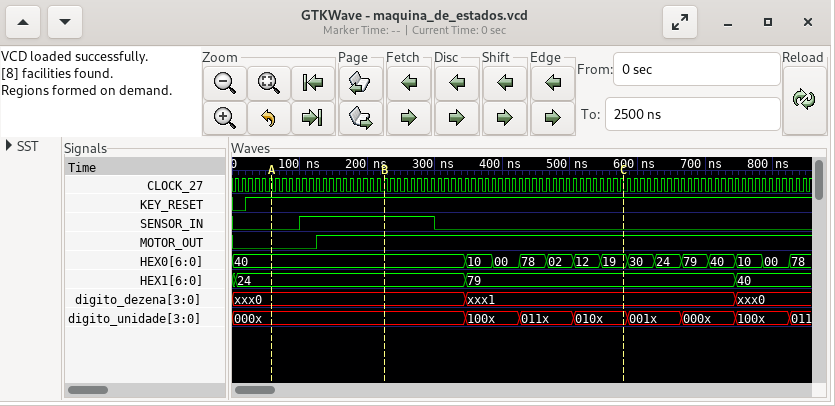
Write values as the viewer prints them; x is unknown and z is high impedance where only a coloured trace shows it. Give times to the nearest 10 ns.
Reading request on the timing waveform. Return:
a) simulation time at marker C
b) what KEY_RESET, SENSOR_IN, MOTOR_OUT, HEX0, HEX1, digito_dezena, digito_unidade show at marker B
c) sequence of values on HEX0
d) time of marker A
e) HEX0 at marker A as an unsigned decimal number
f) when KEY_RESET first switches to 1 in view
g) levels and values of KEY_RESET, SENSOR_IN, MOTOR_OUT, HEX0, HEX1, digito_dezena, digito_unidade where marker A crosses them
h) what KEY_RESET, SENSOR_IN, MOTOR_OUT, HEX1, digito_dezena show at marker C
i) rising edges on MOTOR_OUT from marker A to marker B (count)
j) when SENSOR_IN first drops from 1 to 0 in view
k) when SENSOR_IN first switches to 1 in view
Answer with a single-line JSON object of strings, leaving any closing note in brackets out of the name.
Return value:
{"simulation time at marker C": "580 ns", "what KEY_RESET, SENSOR_IN, MOTOR_OUT, HEX0, HEX1, digito_dezena, digito_unidade show at marker B": "KEY_RESET=1, SENSOR_IN=1, MOTOR_OUT=1, HEX0=40, HEX1=24, digito_dezena=xxx0, digito_unidade=000x", "sequence of values on HEX0": "40, 10, 00, 78, 02, 12, 19, 30, 24, 79, 40, 10, 00, 78", "time of marker A": "60 ns", "HEX0 at marker A as an unsigned decimal number": "64", "when KEY_RESET first switches to 1 in view": "20 ns", "levels and values of KEY_RESET, SENSOR_IN, MOTOR_OUT, HEX0, HEX1, digito_dezena, digito_unidade where marker A crosses them": "KEY_RESET=1, SENSOR_IN=0, MOTOR_OUT=0, HEX0=40, HEX1=24, digito_dezena=xxx0, digito_unidade=000x", "what KEY_RESET, SENSOR_IN, MOTOR_OUT, HEX1, digito_dezena show at marker C": "KEY_RESET=1, SENSOR_IN=0, MOTOR_OUT=1, HEX1=79, digito_dezena=xxx1", "rising edges on MOTOR_OUT from marker A to marker B": "1", "when SENSOR_IN first drops from 1 to 0 in view": "300 ns", "when SENSOR_IN first switches to 1 in view": "100 ns"}
